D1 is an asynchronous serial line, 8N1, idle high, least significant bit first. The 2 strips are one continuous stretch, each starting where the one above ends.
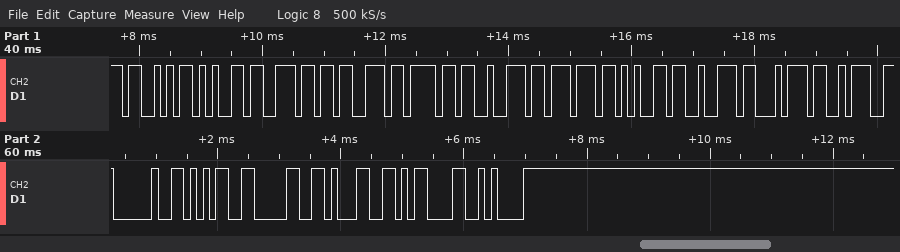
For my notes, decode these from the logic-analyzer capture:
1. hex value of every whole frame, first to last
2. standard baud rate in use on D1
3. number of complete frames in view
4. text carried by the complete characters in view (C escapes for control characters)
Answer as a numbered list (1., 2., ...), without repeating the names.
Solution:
1. 0x53 0x65 0x6E 0x73 0x6F 0x72 0x77 0x65 0x72 0x74 0x3A 0x20 0x35 0x30 0x31 0x0D 0x0A
2. 9600 baud
3. 17
4. "Sensorwert: 501\r\n"
